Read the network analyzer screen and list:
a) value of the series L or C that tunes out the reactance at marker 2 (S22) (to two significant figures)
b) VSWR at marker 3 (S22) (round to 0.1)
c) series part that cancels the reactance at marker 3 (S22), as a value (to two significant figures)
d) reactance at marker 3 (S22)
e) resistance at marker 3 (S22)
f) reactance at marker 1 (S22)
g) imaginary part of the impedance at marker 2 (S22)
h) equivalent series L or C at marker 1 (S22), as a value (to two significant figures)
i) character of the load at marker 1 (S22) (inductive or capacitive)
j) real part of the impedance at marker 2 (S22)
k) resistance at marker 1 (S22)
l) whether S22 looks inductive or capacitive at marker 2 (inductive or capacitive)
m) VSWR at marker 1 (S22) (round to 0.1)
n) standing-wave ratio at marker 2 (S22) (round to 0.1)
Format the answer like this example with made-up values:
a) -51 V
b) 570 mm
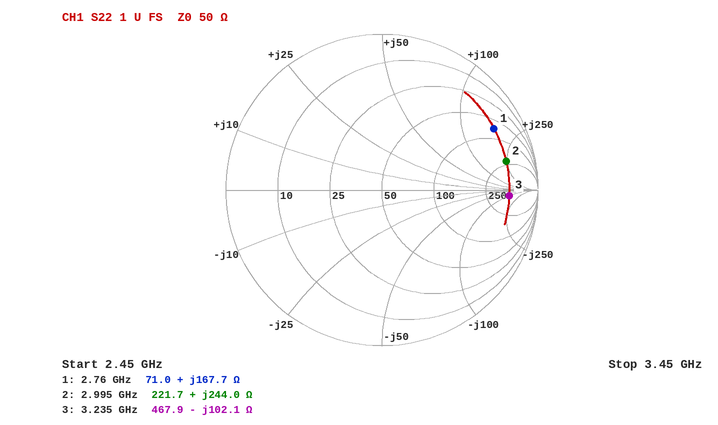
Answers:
a) 220 fF
b) 9.8
c) 5.0 nH
d) -102.1 Ω
e) 467.9 Ω
f) +167.7 Ω
g) +244.0 Ω
h) 9.7 nH
i) inductive
j) 221.7 Ω
k) 71.0 Ω
l) inductive
m) 9.9
n) 9.9
